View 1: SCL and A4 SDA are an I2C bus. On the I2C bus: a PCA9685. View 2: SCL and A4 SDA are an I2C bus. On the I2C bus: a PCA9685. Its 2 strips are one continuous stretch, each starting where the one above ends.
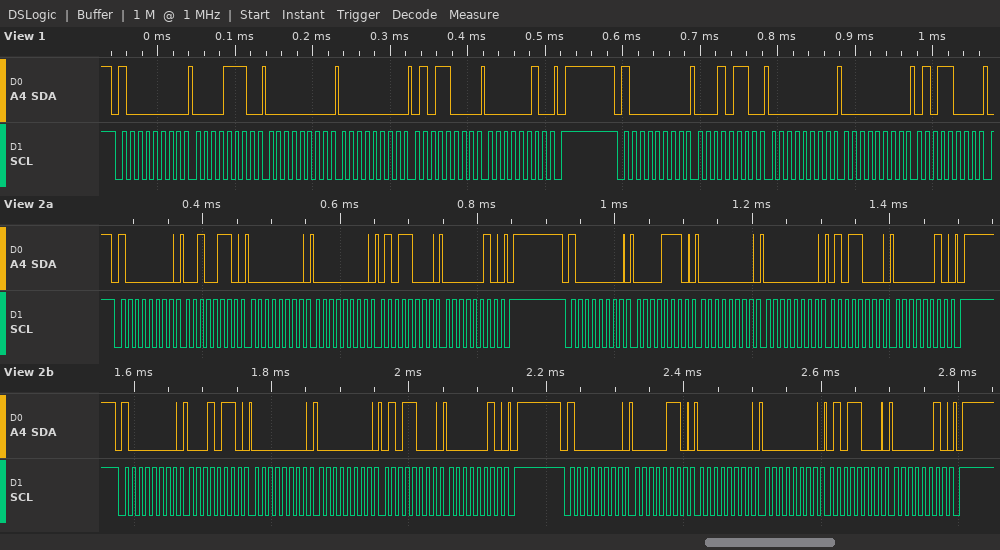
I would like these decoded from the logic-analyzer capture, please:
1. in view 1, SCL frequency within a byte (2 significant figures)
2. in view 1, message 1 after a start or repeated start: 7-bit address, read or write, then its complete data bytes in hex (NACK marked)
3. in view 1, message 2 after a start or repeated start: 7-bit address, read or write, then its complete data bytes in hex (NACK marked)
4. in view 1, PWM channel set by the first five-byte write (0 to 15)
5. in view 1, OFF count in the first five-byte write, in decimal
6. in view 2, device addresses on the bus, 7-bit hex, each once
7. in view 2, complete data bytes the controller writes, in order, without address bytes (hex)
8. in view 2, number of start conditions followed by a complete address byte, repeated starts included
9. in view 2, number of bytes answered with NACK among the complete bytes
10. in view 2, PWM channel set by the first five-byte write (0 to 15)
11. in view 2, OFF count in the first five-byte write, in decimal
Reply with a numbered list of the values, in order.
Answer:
1. 100 kHz
2. 0x40 write: 0E 00 00 58 02
3. 0x40 write: 16 00 00 58
4. 2
5. 600
6. 0x40
7. 26 00 00 58 02 0E 00 00 58 02 16 00 00 58 02 06 00 00 58 02
8. 4
9. 0
10. 8
11. 600
